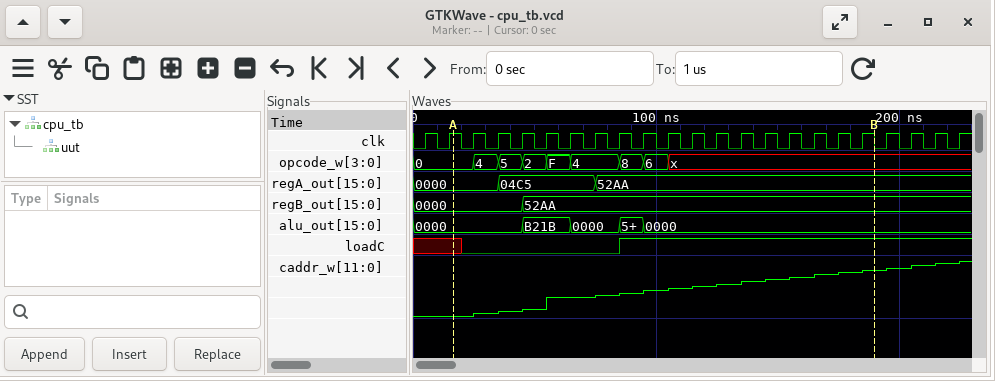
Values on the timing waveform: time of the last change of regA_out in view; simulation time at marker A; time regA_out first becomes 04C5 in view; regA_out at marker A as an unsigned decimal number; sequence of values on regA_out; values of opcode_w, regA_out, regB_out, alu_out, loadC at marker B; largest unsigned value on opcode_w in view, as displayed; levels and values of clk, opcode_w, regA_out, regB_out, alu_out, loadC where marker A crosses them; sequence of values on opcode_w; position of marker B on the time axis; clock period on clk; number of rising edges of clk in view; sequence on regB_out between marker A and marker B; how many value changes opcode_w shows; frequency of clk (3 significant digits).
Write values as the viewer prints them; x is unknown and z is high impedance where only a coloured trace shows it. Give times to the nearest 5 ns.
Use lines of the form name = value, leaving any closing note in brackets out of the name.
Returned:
time of the last change of regA_out in view = 75 ns
simulation time at marker A = 15 ns
time regA_out first becomes 04C5 in view = 35 ns
regA_out at marker A as an unsigned decimal number = 0
sequence of values on regA_out = 0000, 04C5, 52AA
values of opcode_w, regA_out, regB_out, alu_out, loadC at marker B = opcode_w=x, regA_out=52AA, regB_out=52AA, alu_out=0000, loadC=1
largest unsigned value on opcode_w in view, as displayed = F
levels and values of clk, opcode_w, regA_out, regB_out, alu_out, loadC where marker A crosses them = clk=1, opcode_w=0, regA_out=0000, regB_out=0000, alu_out=0000, loadC=x
sequence of values on opcode_w = 0, 4, 5, 2, F, 4, 8, 6, x
position of marker B on the time axis = 190 ns
clock period on clk = 10 ns
number of rising edges of clk in view = 23
sequence on regB_out between marker A and marker B = 0000, 52AA
how many value changes opcode_w shows = 8
frequency of clk = 100 MHz
